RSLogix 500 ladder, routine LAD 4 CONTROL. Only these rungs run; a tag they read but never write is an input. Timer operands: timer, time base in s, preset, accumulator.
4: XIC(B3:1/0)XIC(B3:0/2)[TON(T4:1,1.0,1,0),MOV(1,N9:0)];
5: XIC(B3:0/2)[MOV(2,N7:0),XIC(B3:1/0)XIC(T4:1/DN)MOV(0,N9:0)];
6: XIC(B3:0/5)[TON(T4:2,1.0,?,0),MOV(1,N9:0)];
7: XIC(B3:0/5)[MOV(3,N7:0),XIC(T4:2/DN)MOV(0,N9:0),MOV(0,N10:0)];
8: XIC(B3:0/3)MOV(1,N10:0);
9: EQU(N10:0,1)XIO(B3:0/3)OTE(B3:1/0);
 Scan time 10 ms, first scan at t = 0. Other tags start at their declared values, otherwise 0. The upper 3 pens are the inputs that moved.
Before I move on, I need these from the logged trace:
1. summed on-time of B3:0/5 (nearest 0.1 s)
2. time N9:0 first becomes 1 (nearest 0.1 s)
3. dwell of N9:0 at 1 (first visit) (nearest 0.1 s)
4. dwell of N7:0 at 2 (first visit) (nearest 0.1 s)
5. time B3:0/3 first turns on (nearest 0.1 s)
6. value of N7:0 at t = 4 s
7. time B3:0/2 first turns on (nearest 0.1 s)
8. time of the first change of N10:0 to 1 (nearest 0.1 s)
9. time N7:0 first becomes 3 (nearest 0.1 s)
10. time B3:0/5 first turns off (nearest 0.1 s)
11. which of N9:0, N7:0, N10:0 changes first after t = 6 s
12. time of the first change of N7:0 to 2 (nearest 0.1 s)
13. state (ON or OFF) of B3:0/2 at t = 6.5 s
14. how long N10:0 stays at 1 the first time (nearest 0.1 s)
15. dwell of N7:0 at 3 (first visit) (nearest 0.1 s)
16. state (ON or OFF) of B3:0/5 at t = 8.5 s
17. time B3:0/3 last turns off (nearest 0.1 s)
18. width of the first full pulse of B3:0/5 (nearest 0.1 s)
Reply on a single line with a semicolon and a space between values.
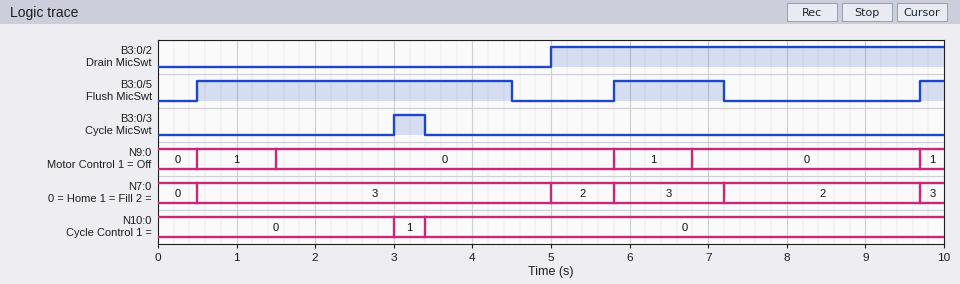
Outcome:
5.7 s; 0.5 s; 1.0 s; 0.8 s; 3.0 s; 3; 5.0 s; 3.0 s; 0.5 s; 4.5 s; N9:0; 5.0 s; ON; 0.4 s; 4.5 s; OFF; 3.4 s; 4.0 s
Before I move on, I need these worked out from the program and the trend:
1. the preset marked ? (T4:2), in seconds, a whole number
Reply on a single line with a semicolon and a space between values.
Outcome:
1 s
